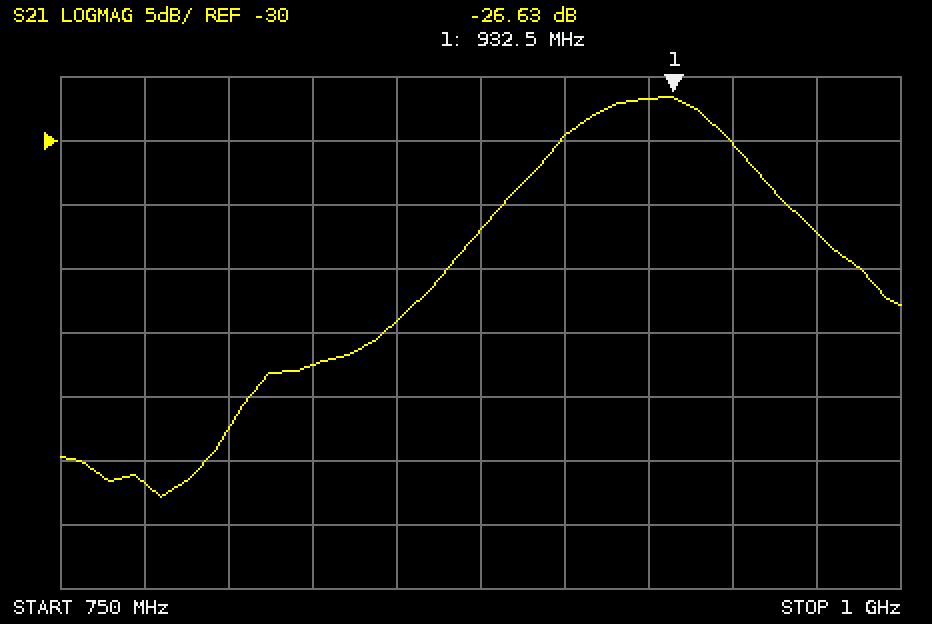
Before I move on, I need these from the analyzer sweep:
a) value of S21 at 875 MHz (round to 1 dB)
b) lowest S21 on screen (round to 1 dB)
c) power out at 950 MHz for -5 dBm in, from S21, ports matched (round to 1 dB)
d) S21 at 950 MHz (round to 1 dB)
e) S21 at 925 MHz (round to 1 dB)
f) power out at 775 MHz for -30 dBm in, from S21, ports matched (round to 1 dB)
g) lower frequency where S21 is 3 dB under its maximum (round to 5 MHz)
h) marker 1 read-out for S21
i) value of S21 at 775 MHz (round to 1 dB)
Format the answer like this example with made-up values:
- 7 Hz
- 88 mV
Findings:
- -37 dB
- -58 dB
- -35 dBm
- -30 dB
- -27 dB
- -87 dBm
- 900 MHz
- -26.63 dB
- -57 dB
